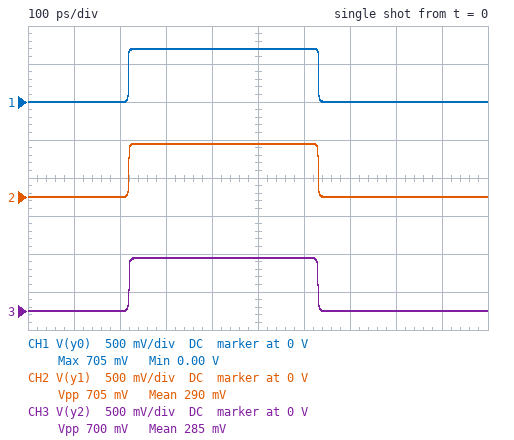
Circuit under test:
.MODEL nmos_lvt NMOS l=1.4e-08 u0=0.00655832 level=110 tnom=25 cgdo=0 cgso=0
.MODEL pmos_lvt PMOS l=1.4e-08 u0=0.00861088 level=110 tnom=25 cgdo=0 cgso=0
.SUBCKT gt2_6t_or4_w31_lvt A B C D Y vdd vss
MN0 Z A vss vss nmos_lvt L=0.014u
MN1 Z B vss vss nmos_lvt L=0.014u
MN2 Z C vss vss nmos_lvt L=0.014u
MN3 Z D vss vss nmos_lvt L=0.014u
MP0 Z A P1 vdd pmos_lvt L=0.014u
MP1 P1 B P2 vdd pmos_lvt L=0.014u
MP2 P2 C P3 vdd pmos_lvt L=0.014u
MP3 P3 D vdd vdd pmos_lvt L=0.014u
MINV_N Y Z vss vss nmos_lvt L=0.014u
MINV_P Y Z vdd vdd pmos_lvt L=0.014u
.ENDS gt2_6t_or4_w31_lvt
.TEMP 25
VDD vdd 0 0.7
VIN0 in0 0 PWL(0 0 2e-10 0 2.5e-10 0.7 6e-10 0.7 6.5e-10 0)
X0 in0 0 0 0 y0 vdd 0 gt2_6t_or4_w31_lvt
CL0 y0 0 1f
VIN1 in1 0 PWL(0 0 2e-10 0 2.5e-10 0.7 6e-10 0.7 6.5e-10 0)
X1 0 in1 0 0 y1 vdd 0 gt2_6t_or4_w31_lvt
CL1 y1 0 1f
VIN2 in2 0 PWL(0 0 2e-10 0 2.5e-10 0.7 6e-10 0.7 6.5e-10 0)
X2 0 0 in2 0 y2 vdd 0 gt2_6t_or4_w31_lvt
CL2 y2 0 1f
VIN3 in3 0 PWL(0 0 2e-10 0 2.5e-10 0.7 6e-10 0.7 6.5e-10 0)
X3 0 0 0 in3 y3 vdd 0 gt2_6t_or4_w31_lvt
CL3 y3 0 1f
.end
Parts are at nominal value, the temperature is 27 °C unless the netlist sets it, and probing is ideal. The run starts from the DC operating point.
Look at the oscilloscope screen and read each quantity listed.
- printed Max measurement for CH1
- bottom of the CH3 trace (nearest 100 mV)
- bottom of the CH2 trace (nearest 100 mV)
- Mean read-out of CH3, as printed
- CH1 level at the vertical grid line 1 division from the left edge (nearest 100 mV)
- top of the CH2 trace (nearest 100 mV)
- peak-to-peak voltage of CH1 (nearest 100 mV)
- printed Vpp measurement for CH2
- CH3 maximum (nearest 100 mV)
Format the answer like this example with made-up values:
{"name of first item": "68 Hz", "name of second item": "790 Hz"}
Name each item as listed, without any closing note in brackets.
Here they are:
{"printed Max measurement for CH1": "705 mV", "bottom of the CH3 trace": "0 V", "bottom of the CH2 trace": "0 V", "Mean read-out of CH3, as printed": "285 mV", "CH1 level at the vertical grid line 1 division from the left edge": "0 V", "top of the CH2 trace": "700 mV", "peak-to-peak voltage of CH1": "700 mV", "printed Vpp measurement for CH2": "705 mV", "CH3 maximum": "700 mV"}
